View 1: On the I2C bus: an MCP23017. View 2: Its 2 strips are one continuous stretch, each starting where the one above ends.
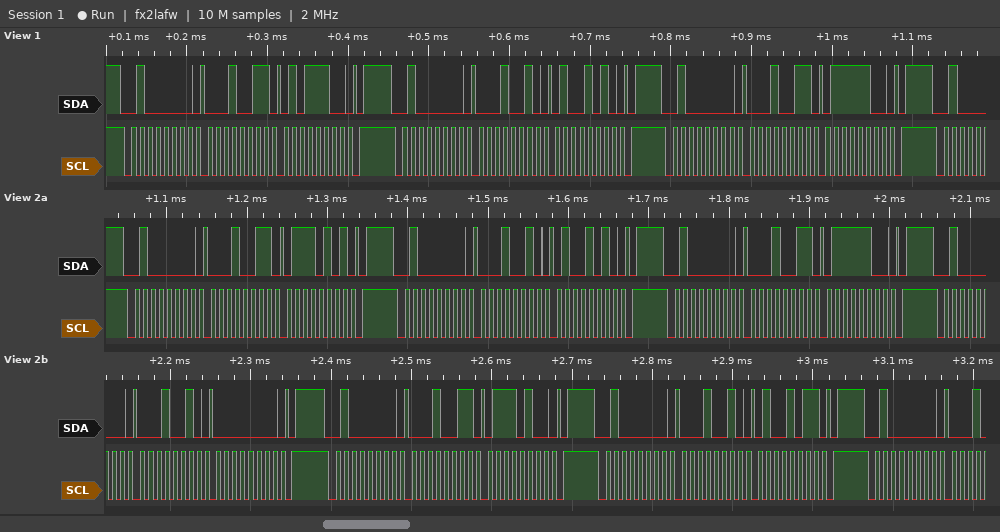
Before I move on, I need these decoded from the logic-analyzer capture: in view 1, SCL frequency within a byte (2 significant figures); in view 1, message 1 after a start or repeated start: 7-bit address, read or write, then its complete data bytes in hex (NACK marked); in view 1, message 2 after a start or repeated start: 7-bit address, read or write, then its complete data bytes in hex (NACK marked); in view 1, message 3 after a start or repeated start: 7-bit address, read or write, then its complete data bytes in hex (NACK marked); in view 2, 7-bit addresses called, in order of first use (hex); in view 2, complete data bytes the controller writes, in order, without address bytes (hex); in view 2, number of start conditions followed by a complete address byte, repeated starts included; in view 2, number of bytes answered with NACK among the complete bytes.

100 kHz
0x20 write: 13 5C
0x20 write: 12 4A
0x20 write: 13 7C
0x20
13 75 12 4A 13 7C 12 00 13 74 12 4B
7
0
